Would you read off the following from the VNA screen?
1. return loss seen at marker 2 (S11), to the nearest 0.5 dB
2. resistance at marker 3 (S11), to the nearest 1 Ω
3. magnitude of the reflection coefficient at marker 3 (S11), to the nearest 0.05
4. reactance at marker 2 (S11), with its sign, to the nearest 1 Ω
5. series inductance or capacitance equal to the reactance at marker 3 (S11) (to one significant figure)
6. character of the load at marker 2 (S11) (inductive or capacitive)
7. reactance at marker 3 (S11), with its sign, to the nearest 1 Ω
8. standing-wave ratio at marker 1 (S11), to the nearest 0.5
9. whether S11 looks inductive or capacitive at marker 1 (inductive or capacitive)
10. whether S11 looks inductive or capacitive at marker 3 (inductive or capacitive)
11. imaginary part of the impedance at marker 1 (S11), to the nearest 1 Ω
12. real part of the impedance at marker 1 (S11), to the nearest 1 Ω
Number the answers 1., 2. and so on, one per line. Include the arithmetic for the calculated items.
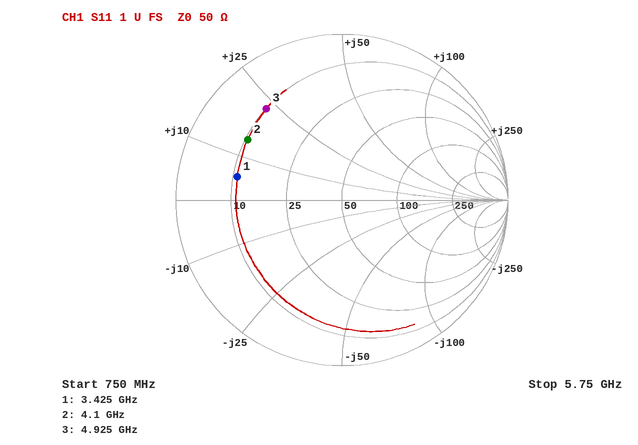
1. 3.5 dB
2. 10 Ω
3. 0.70
4. +14 Ω
5. L = 23 Ω/(2π × 4.925 GHz) ≈ 743 pH, so 700 pH to one significant figure
6. inductive
7. +23 Ω
8. 4.5
9. inductive
10. inductive
11. +5 Ω
12. 11 Ω
